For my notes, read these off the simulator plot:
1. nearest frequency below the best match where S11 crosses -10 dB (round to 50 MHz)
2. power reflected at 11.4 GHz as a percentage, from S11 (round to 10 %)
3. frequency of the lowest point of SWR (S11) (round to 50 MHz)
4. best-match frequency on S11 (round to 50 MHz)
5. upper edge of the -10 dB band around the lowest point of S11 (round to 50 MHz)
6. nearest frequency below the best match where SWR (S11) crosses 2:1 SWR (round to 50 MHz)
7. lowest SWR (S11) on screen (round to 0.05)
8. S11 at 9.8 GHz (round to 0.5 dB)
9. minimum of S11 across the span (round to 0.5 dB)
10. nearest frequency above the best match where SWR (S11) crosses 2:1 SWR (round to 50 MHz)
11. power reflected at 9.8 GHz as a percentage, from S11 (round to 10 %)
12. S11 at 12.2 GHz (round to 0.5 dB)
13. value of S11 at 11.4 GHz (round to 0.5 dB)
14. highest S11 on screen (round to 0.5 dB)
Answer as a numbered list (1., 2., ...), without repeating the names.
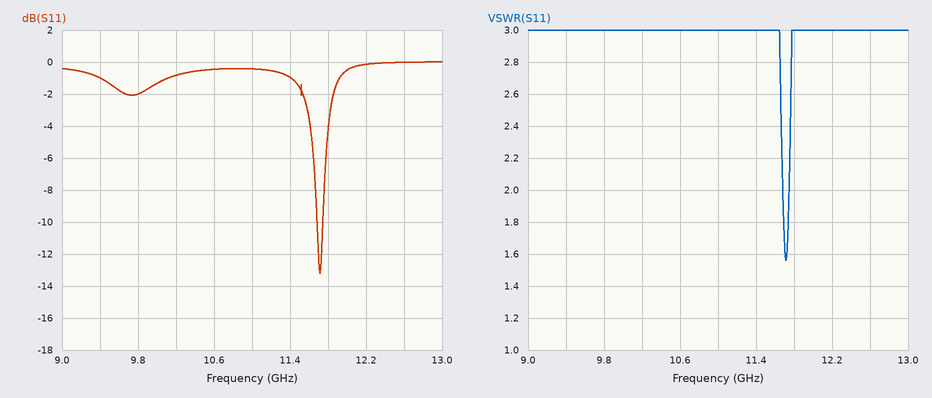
1. 11.70 GHz
2. 80 %
3. 11.70 GHz
4. 11.70 GHz
5. 11.75 GHz
6. 11.70 GHz
7. 1.55
8. -2.0 dB
9. -13.0 dB
10. 11.75 GHz
11. 60 %
12. 0.0 dB
13. -1.0 dB
14. 0.0 dB
